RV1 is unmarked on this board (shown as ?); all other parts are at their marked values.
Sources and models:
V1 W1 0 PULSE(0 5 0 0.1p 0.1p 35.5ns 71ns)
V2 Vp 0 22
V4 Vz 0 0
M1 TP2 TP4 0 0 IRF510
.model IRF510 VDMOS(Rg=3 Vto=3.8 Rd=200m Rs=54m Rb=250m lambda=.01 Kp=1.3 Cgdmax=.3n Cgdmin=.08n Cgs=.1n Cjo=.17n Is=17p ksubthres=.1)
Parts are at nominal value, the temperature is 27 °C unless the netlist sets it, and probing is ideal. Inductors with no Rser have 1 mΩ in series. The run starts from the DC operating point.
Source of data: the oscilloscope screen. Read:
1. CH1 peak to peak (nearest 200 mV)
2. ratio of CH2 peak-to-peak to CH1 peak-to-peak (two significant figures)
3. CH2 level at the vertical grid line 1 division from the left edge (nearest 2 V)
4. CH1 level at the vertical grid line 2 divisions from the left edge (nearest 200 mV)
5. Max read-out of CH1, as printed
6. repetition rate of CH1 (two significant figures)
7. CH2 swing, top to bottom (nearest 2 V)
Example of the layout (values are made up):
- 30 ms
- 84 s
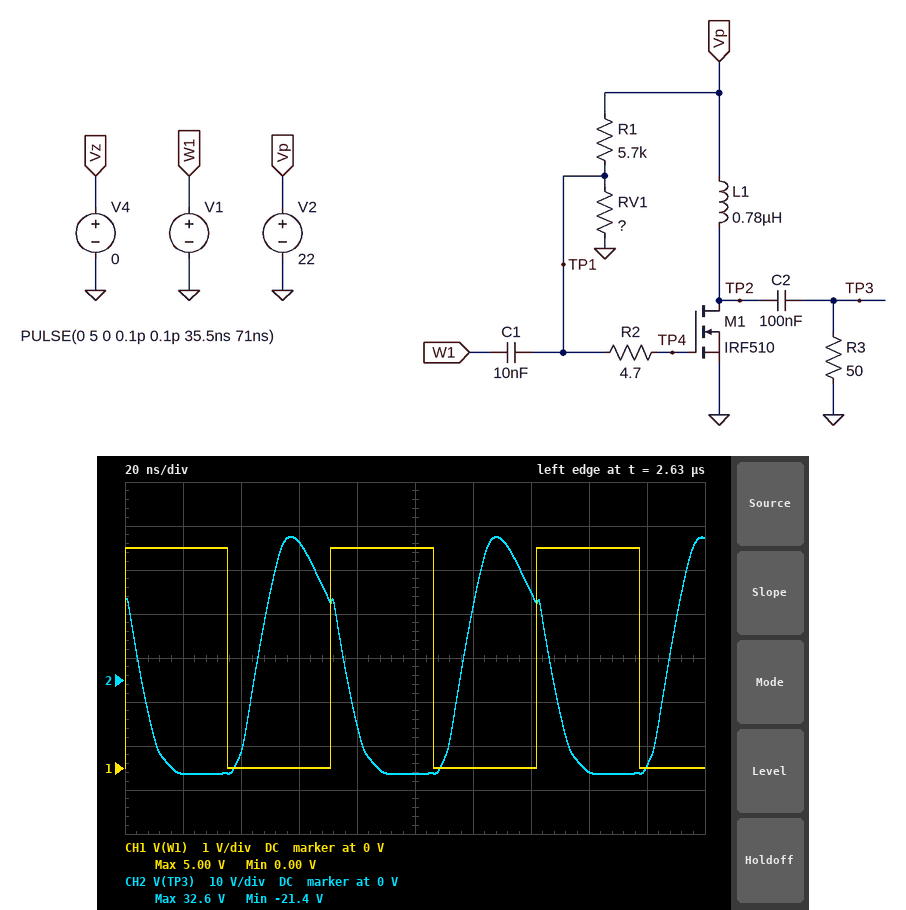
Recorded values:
- 5.0 V
- 11
- -22 V
- 0 V
- 5.00 V
- 14 MHz
- 54 V
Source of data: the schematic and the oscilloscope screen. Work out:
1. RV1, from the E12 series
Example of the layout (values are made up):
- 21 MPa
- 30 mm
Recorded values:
- 820 Ω
